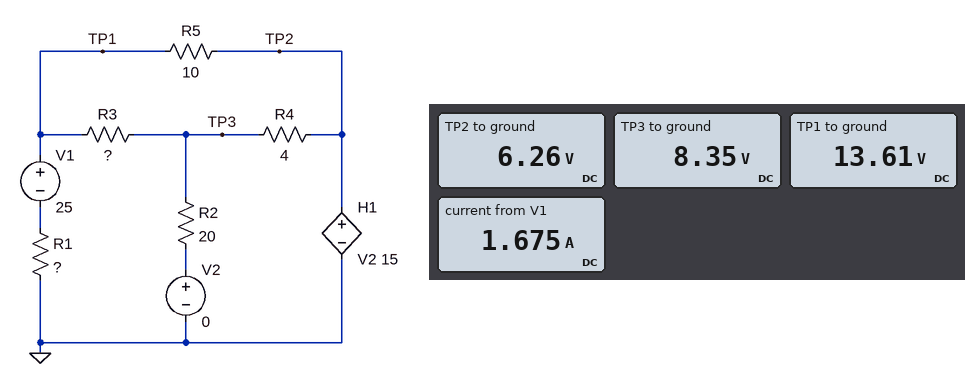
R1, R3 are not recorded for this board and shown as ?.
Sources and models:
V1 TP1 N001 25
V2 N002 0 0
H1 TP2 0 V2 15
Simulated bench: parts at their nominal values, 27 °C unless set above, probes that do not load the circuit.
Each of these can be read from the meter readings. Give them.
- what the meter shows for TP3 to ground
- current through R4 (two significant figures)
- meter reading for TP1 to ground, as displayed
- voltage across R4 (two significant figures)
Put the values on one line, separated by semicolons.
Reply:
8.35 V; 520 mA; 13.61 V; 2.1 V
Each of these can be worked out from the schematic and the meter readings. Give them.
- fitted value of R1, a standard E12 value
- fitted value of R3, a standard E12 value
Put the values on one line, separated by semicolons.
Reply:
6.8 Ω; 5.6 Ω
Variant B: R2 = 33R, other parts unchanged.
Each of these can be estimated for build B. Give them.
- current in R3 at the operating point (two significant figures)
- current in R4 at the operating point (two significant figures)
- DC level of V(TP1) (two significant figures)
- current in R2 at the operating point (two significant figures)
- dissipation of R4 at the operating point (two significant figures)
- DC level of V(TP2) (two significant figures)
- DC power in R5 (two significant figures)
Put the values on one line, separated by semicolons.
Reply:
1.0 A; 840 mA; 12 V; 190 mA; 2.8 W; 2.8 V; 8.2 W
